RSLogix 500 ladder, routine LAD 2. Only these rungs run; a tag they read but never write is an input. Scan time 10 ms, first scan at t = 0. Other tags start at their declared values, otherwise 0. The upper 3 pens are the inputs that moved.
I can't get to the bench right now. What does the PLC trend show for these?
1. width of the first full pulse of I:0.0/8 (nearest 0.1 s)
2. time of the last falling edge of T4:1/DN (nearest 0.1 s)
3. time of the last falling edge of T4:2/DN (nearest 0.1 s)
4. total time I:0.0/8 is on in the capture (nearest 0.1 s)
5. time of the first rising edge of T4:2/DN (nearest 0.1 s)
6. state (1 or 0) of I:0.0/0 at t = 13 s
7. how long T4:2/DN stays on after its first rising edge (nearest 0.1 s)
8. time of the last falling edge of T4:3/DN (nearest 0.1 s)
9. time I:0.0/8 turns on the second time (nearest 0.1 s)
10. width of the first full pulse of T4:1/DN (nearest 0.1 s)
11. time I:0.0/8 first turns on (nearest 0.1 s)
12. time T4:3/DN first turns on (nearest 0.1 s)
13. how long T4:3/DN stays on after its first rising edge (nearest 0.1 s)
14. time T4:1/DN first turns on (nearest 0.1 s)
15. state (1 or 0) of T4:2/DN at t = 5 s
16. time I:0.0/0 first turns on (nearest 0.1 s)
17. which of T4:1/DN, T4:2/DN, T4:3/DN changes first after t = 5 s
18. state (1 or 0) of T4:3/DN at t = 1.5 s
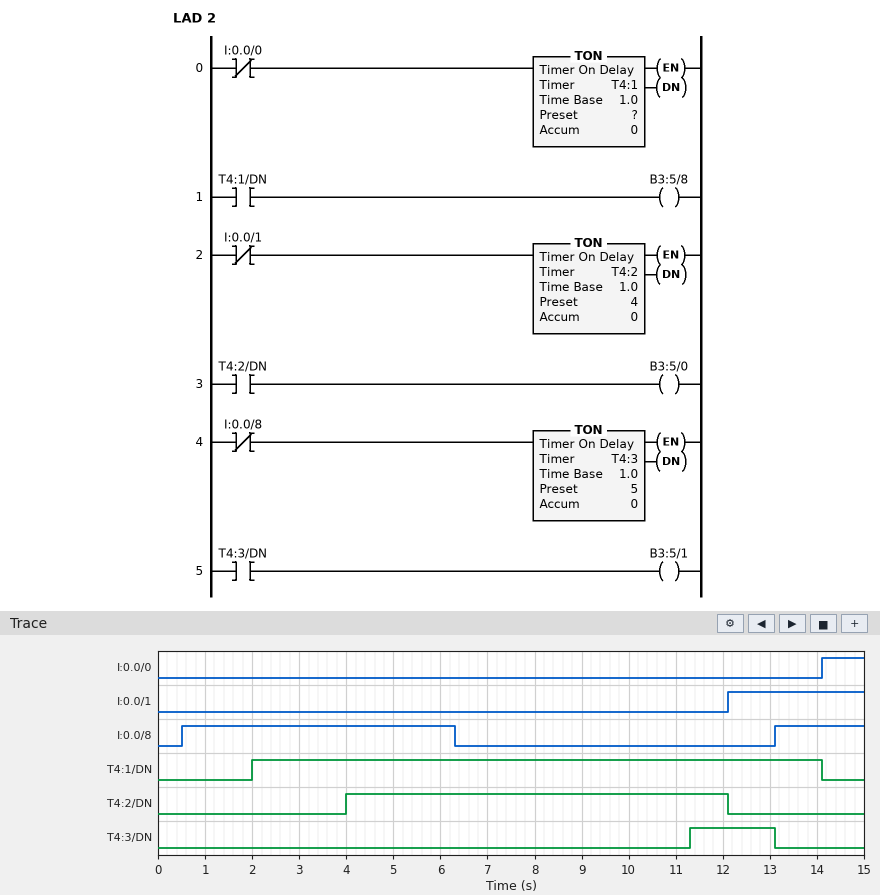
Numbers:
5.8 s
14.1 s
12.1 s
7.7 s
4.0 s
0
8.1 s
13.1 s
13.1 s
12.1 s
0.5 s
11.3 s
1.8 s
2.0 s
1
14.1 s
T4:3/DN
0
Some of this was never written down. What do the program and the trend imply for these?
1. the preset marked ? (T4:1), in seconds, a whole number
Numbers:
2 s
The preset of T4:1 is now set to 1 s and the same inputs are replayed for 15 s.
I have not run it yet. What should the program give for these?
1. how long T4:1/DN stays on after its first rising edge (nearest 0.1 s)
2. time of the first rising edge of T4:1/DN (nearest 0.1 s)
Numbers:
13.1 s
1.0 s
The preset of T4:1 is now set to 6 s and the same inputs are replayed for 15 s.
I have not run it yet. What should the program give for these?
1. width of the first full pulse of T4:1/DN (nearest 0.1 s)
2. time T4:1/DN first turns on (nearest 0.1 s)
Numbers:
8.1 s
6.0 s
